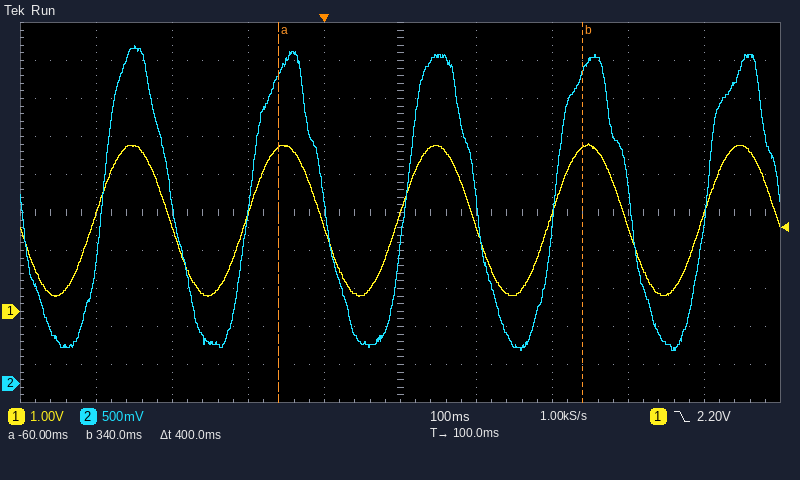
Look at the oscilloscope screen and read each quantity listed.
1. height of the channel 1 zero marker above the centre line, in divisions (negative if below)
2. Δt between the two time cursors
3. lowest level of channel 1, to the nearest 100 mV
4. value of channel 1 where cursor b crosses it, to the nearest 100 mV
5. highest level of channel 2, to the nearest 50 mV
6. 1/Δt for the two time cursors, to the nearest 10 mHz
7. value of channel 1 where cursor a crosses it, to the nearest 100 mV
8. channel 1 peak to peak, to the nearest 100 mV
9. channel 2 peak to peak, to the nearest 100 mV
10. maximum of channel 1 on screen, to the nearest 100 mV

-2.6 div
400 ms
400 mV
4.3 V
4.45 V
2.50 Hz
4.3 V
4.0 V
4.00 V
4.4 V
